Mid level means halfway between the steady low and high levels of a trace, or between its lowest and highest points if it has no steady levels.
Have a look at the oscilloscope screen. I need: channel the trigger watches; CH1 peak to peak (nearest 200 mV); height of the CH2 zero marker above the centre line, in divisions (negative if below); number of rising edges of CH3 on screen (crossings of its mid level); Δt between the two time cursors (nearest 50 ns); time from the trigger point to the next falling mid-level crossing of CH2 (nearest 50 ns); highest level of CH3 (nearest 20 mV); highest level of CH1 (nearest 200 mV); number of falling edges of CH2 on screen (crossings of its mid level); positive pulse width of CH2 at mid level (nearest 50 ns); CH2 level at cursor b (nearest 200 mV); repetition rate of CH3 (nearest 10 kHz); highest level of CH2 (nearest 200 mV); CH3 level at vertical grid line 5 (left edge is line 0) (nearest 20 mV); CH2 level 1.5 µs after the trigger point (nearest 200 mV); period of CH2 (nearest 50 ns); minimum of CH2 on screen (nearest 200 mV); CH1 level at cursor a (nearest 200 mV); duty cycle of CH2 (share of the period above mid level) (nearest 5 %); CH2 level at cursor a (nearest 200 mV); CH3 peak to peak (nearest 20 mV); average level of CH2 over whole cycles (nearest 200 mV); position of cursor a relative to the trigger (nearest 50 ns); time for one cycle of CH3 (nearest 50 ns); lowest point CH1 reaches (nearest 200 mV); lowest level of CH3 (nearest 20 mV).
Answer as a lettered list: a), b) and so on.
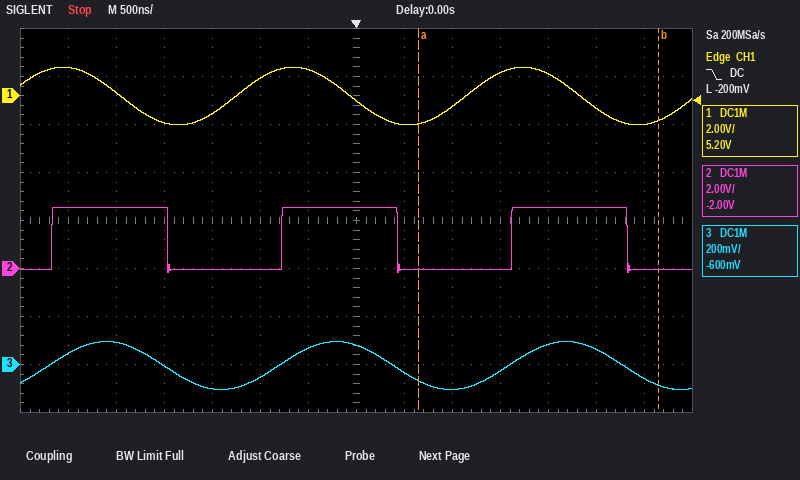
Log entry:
a) CH1
b) 2.4 V
c) -1.0 div
d) 3
e) 2.50 µs
f) 450 ns
g) 100 mV
h) 1.2 V
i) 3
j) 1.20 µs
k) 0.0 V
l) 420 kHz
m) 2.6 V
n) -60 mV
o) 0.0 V
p) 2.40 µs
q) -200 mV
r) -1.2 V
s) 50 %
t) 0.0 V
u) 200 mV
v) 1.2 V
w) +650 ns
x) 2.40 µs
y) -1.2 V
z) -100 mV
